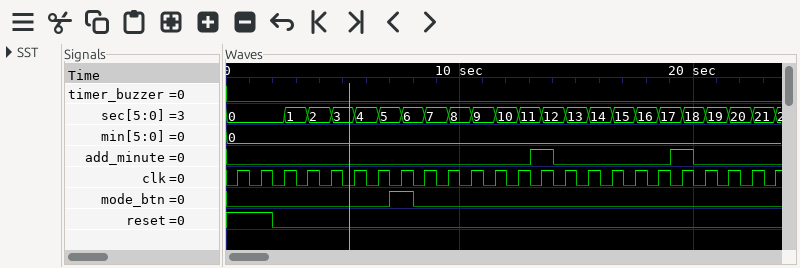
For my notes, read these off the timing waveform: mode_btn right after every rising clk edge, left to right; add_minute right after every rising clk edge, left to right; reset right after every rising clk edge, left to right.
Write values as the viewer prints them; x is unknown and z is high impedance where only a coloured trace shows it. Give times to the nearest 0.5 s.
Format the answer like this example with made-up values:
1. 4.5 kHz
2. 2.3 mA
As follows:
1. 0 0 0 0 0 0 0 1 0 0 0 0 0 0 0 0 0 0 0 0 0 0 0 0
2. 0 0 0 0 0 0 0 0 0 0 0 0 0 1 0 0 0 0 0 1 0 0 0 0
3. 1 1 0 0 0 0 0 0 0 0 0 0 0 0 0 0 0 0 0 0 0 0 0 0
